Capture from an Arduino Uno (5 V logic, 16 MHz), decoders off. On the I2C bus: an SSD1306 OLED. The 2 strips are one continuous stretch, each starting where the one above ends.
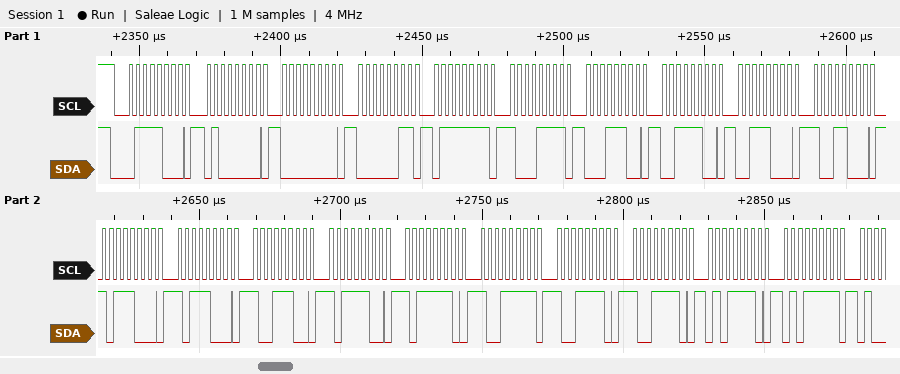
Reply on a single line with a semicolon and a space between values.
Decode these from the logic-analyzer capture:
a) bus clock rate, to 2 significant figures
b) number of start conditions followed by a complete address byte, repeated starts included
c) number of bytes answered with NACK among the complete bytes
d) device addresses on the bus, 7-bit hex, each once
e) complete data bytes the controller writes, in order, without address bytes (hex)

400 kHz; 1; 0; 0x3C; 40 00 03 7F 8F 1C 3C 38 98 B8 B8 9C BC BE 9F 9E 9E 5E 5F
